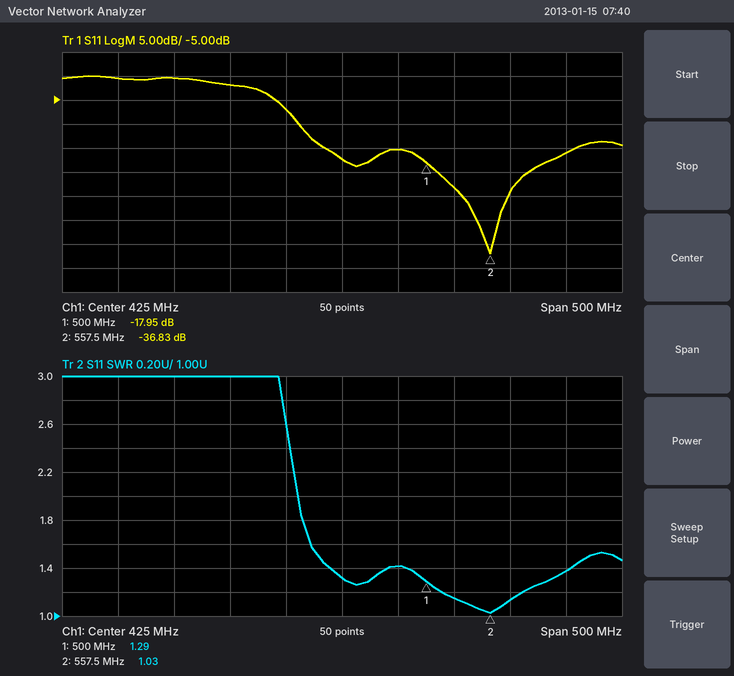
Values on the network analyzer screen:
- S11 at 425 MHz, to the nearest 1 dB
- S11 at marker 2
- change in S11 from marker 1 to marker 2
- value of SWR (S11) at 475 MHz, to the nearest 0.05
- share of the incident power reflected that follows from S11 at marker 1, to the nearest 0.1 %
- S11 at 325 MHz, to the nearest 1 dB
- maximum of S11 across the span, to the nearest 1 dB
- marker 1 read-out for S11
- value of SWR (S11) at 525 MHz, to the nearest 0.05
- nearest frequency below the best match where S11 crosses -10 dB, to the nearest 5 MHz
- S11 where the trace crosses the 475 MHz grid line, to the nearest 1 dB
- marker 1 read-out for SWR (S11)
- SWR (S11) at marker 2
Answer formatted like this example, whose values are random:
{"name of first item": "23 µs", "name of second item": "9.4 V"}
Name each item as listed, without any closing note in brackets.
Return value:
{"S11 at 425 MHz, to the nearest 1 dB": "-17 dB", "S11 at marker 2": "-36.83 dB", "change in S11 from marker 1 to marker 2": "-18.88 dB", "value of SWR (S11) at 475 MHz, to the nearest 0.05": "1.40", "share of the incident power reflected that follows from S11 at marker 1, to the nearest 0.1 %": "1.6 %", "S11 at 325 MHz, to the nearest 1 dB": "-2 dB", "maximum of S11 across the span, to the nearest 1 dB": "0 dB", "marker 1 read-out for S11": "-17.95 dB", "value of SWR (S11) at 525 MHz, to the nearest 0.05": "1.15", "nearest frequency below the best match where S11 crosses -10 dB, to the nearest 5 MHz": "385 MHz", "S11 where the trace crosses the 475 MHz grid line, to the nearest 1 dB": "-15 dB", "marker 1 read-out for SWR": "1.29", "SWR (S11) at marker 2": "1.03"}
